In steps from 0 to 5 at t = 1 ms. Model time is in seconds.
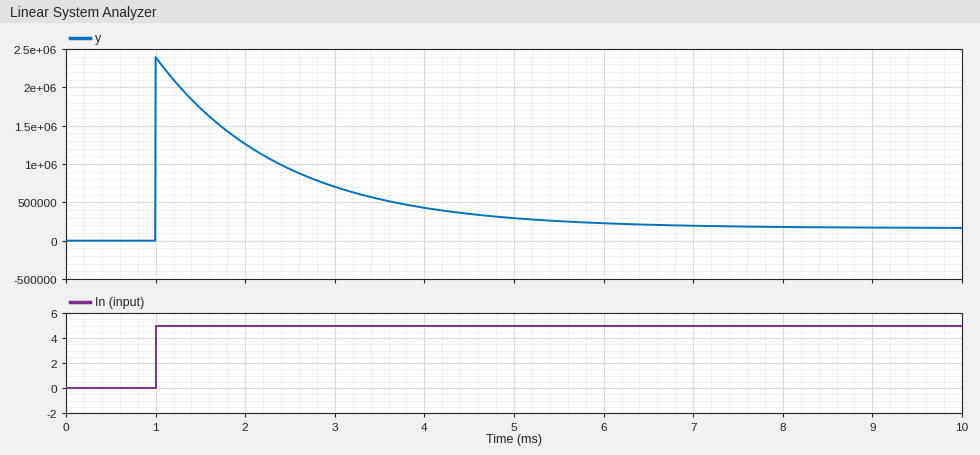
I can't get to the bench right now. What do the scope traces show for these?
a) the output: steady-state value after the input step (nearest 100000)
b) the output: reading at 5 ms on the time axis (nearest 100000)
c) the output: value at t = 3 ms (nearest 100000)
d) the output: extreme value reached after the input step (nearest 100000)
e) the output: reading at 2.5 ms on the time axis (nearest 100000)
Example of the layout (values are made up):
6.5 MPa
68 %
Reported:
200000
300000
700000
2400000
900000
